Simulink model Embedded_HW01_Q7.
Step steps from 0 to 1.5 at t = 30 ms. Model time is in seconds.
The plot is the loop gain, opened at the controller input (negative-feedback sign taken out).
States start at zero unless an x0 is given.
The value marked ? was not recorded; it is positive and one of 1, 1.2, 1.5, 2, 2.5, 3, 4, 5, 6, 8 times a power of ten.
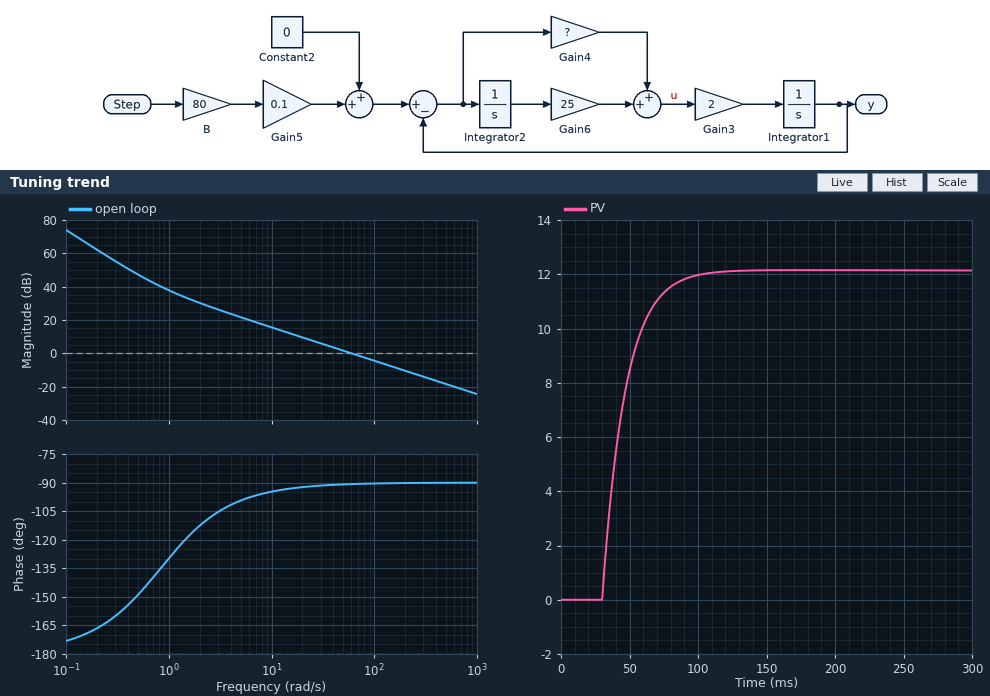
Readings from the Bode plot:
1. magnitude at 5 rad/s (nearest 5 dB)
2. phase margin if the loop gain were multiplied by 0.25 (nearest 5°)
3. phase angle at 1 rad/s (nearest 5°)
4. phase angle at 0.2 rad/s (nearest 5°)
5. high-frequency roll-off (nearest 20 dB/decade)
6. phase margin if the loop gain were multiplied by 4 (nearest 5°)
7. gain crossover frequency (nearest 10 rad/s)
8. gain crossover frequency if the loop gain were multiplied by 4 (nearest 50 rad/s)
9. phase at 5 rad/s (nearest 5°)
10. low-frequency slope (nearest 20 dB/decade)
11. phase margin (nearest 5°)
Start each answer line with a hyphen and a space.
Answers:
- 20 dB
- 85°
- -130°
- -165°
- -20 dB/decade
- 90°
- 60 rad/s
- 250 rad/s
- -100°
- -40 dB/decade
- 90°
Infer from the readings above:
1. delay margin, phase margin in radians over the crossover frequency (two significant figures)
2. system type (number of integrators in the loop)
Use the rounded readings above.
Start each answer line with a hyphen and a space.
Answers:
- 0.026 s
- 2
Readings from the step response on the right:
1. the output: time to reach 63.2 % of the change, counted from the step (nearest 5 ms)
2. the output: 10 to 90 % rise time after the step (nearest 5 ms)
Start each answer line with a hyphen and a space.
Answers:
- 15 ms
- 35 ms
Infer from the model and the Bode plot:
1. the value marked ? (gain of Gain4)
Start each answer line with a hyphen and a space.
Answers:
- 30
